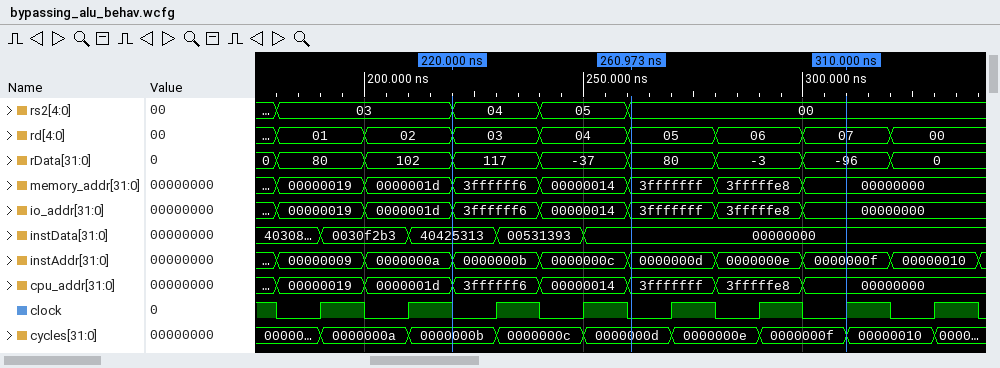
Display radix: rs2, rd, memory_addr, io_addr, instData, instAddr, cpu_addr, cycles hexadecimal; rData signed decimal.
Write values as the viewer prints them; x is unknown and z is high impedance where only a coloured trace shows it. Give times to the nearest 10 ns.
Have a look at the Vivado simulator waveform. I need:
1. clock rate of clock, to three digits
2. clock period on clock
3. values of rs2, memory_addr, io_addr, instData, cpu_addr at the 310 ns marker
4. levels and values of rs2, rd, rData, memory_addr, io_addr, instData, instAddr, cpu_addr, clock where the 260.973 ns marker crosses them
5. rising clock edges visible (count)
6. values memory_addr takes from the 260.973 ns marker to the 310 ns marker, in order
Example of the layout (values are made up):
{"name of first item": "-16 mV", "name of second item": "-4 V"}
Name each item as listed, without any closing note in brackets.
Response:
{"clock rate of clock, to three digits": "50.0 MHz", "clock period on clock": "20 ns", "values of rs2, memory_addr, io_addr, instData, cpu_addr at the 310 ns marker": "rs2=00, memory_addr=00000000, io_addr=00000000, instData=00000000, cpu_addr=00000000", "levels and values of rs2, rd, rData, memory_addr, io_addr, instData, instAddr, cpu_addr, clock where the 260.973 ns marker crosses them": "rs2=00, rd=05, rData=80, memory_addr=3fffffff, io_addr=3fffffff, instData=00000000, instAddr=0000000d, cpu_addr=3fffffff, clock=0", "rising clock edges visible": "8", "values memory_addr takes from the 260.973 ns marker to the 310 ns marker, in order": "3fffffff, 3fffffe8, 00000000"}
